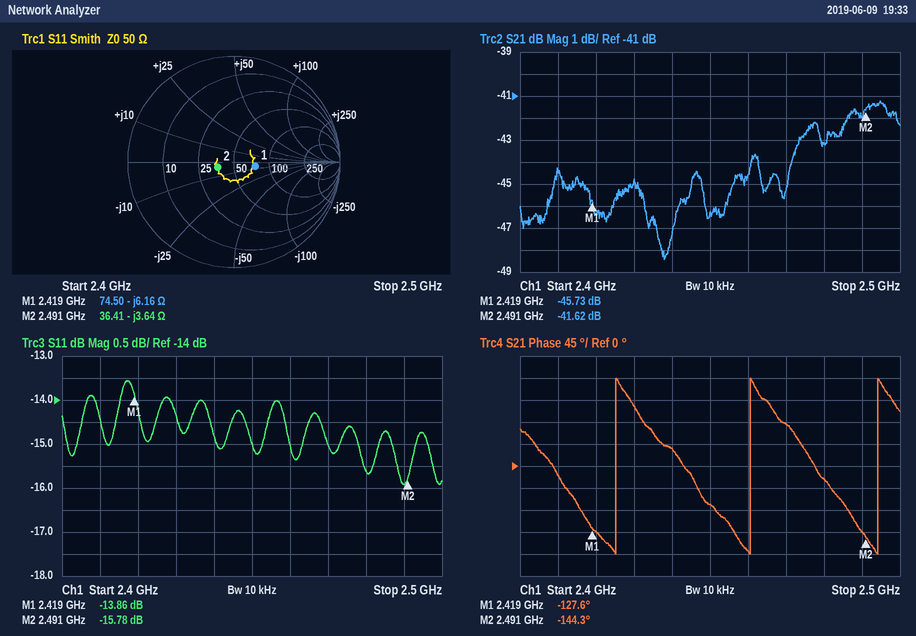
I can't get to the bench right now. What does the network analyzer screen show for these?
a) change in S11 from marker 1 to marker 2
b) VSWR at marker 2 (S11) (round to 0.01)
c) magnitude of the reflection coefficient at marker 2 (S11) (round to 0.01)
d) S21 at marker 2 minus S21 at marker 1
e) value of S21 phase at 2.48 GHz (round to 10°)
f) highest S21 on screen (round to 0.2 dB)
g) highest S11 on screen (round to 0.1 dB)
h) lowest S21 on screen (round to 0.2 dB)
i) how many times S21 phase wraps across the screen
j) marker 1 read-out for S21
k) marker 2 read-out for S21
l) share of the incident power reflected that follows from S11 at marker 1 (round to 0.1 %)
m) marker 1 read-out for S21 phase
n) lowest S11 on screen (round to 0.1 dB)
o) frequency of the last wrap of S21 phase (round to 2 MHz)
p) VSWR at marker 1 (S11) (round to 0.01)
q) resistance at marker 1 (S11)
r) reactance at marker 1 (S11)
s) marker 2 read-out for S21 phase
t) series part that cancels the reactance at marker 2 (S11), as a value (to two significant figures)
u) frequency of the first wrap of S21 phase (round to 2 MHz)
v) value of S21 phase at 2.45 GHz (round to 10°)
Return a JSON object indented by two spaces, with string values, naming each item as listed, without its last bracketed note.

{
  "change in S11 from marker 1 to marker 2": "-1.92 dB",
  "VSWR at marker 2 (S11)": "1.39",
  "magnitude of the reflection coefficient at marker 2 (S11)": "0.16",
  "S21 at marker 2 minus S21 at marker 1": "4.11 dB",
  "value of S21 phase at 2.48 GHz": "-30°",
  "highest S21 on screen": "-41.2 dB",
  "highest S11 on screen": "-13.6 dB",
  "lowest S21 on screen": "-48.4 dB",
  "how many times S21 phase wraps across the screen": "3",
  "marker 1 read-out for S21": "-45.73 dB",
  "marker 2 read-out for S21": "-41.62 dB",
  "share of the incident power reflected that follows from S11 at marker 1": "4.1 %",
  "marker 1 read-out for S21 phase": "-127.6°",
  "lowest S11 on screen": "-15.9 dB",
  "frequency of the last wrap of S21 phase": "2.494 GHz",
  "VSWR at marker 1 (S11)": "1.51",
  "resistance at marker 1": "74.50 Ω",
  "reactance at marker 1": "-6.16 Ω",
  "marker 2 read-out for S21 phase": "-144.3°",
  "series part that cancels the reactance at marker 2 (S11), as a value": "230 pH",
  "frequency of the first wrap of S21 phase": "2.426 GHz",
  "value of S21 phase at 2.45 GHz": "-80°"
}
